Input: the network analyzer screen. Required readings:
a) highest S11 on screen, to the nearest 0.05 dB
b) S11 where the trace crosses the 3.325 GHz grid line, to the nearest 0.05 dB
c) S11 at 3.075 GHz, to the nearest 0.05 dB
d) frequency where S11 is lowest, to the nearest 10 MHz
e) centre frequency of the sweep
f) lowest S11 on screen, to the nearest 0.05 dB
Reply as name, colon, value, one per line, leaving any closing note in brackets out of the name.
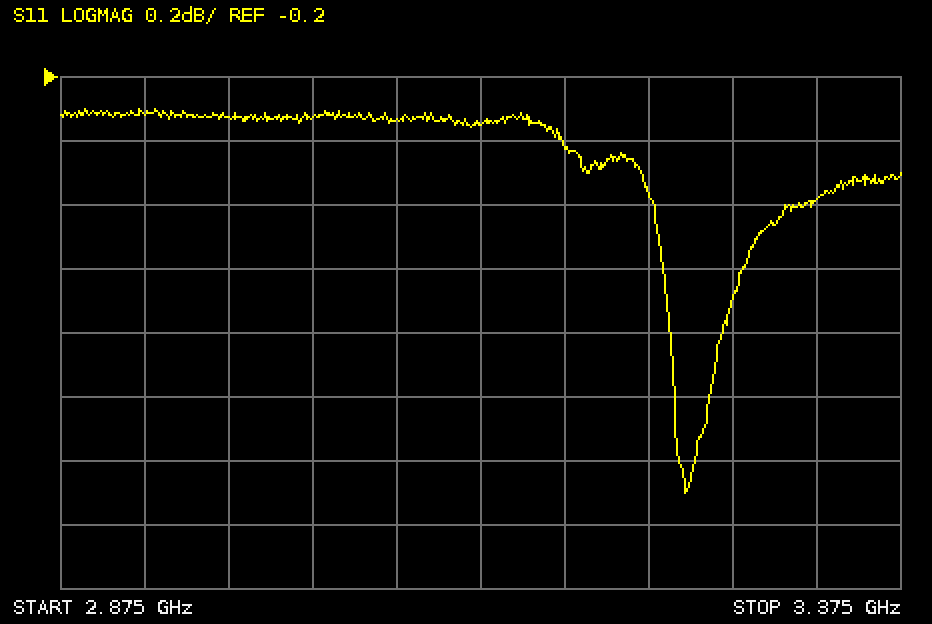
highest S11 on screen, to the nearest 0.05 dB: -0.30 dB
S11 where the trace crosses the 3.325 GHz grid line, to the nearest 0.05 dB: -0.60 dB
S11 at 3.075 GHz, to the nearest 0.05 dB: -0.35 dB
frequency where S11 is lowest, to the nearest 10 MHz: 3.25 GHz
centre frequency of the sweep: 3.125 GHz
lowest S11 on screen, to the nearest 0.05 dB: -1.50 dB
